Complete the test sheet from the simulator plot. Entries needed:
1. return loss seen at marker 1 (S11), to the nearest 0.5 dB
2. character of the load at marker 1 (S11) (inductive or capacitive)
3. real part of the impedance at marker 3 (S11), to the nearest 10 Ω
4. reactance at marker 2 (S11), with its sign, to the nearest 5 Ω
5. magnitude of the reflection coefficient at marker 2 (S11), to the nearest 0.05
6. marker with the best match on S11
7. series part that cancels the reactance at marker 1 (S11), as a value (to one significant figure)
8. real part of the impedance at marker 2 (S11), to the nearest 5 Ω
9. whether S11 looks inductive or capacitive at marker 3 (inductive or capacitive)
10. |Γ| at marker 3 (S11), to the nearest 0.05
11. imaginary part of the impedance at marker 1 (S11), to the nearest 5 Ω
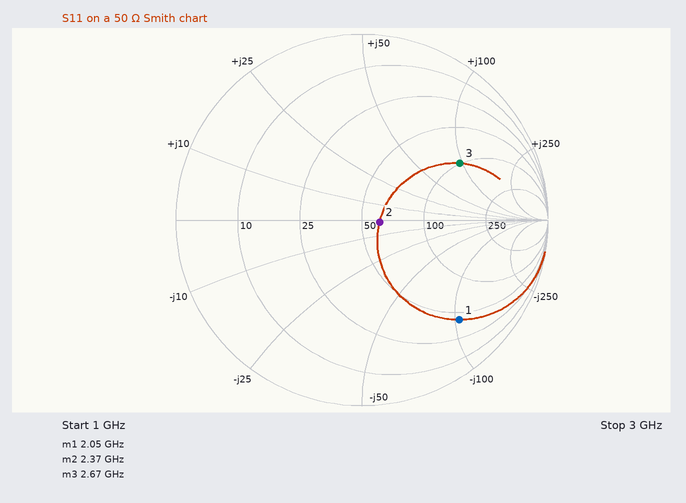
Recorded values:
2.5 dB
capacitive
100 Ω
0 Ω
0.10
marker 2
8 nH
60 Ω
inductive
0.60
-105 Ω
